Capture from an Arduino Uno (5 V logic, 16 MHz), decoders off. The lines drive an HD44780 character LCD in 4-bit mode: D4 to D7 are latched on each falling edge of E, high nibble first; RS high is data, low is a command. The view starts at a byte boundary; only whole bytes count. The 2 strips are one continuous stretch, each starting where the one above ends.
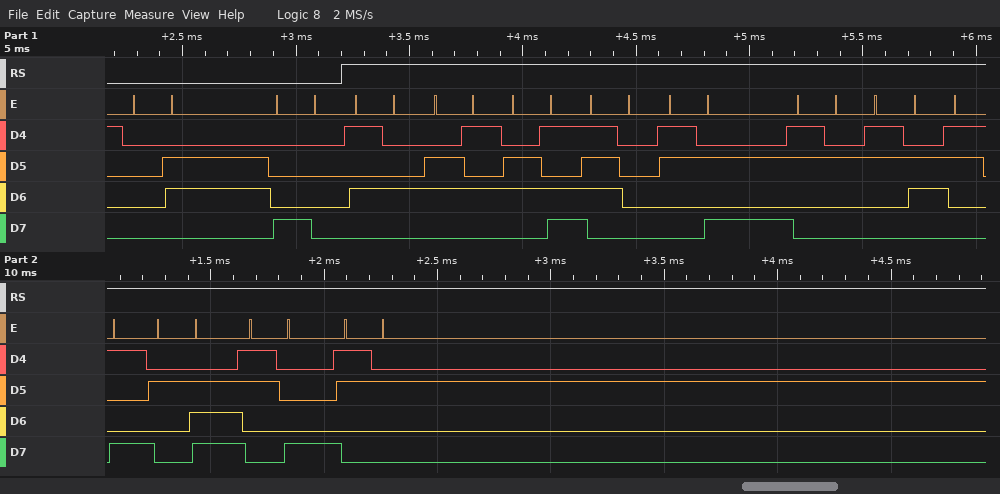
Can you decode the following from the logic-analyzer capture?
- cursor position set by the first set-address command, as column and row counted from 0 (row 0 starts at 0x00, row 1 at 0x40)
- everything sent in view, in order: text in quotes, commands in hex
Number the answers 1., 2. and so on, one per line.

1. column 0, row 0
2. 0x06 0x80 "Temp:269.82"
